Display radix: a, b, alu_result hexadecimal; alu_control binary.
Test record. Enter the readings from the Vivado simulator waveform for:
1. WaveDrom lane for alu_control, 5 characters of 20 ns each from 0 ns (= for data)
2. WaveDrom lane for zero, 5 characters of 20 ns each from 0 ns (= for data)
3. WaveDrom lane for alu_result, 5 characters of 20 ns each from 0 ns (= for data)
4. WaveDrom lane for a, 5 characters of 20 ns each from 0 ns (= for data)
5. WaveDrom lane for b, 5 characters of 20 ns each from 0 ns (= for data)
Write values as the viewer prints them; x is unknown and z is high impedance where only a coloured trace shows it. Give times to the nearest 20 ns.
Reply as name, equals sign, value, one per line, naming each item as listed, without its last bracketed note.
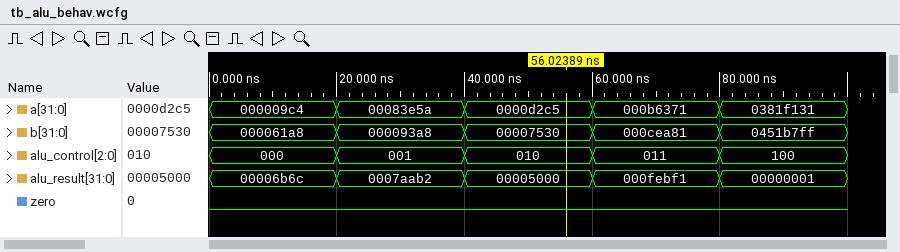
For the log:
WaveDrom lane for alu_control, 5 characters of 20 ns each from 0 ns = {name: 'alu_control', wave: '=====', data: '000 001 010 011 100'}
WaveDrom lane for zero, 5 characters of 20 ns each from 0 ns = {name: 'zero', wave: '0....'}
WaveDrom lane for alu_result, 5 characters of 20 ns each from 0 ns = {name: 'alu_result', wave: '=====', data: '00006b6c 0007aab2 00005000 000febf1 00000001'}
WaveDrom lane for a, 5 characters of 20 ns each from 0 ns = {name: 'a', wave: '=====', data: '000009c4 00083e5a 0000d2c5 000b6371 0381f131'}
WaveDrom lane for b, 5 characters of 20 ns each from 0 ns = {name: 'b', wave: '=====', data: '000061a8 000093a8 00007530 000cea81 0451b7ff'}
